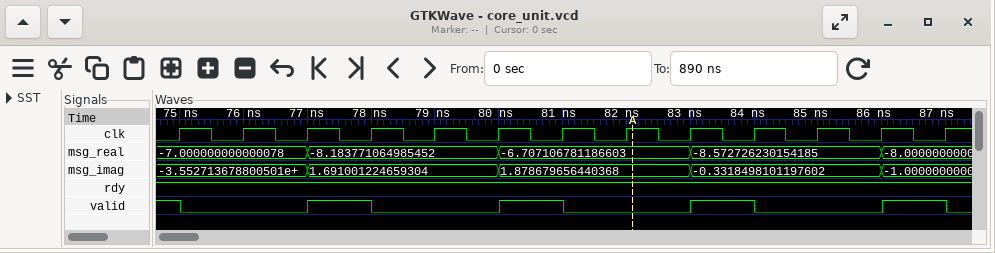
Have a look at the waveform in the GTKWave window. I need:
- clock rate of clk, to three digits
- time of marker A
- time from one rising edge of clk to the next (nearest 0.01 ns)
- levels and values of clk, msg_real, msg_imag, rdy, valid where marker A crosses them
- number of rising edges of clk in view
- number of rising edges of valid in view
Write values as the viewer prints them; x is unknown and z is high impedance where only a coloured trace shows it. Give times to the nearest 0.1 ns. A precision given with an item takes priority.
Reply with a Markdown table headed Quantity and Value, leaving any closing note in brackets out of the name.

| Quantity | Value |
|---|---|
| clock rate of clk, to three digits | 1.00 GHz |
| time of marker A | 82.1 ns |
| time from one rising edge of clk to the next | 1 ns |
| levels and values of clk, msg_real, msg_imag, rdy, valid where marker A crosses them | clk=1, msg_real=-6.707106781186603, msg_imag=1.878679656440368, rdy=1, valid=0 |
| number of rising edges of clk in view | 13 |
| number of rising edges of valid in view | 4 |
